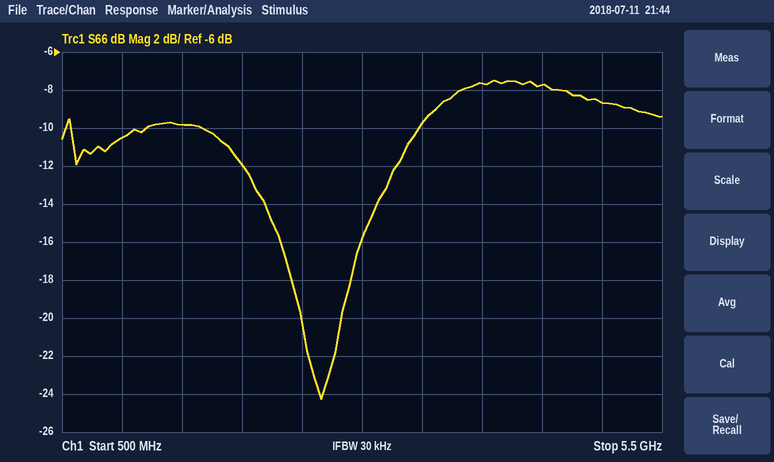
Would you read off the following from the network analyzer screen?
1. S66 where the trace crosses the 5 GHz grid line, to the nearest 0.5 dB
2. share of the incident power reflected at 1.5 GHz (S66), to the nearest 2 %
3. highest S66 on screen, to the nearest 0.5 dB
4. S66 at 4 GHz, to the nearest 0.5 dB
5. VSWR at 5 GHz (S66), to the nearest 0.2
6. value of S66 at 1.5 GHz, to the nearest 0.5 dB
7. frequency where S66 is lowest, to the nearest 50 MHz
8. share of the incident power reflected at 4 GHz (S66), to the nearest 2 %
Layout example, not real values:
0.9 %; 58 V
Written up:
-8.5 dB; 10 %; -7.5 dB; -7.5 dB; 2.2; -10.0 dB; 2.65 GHz; 18 %
